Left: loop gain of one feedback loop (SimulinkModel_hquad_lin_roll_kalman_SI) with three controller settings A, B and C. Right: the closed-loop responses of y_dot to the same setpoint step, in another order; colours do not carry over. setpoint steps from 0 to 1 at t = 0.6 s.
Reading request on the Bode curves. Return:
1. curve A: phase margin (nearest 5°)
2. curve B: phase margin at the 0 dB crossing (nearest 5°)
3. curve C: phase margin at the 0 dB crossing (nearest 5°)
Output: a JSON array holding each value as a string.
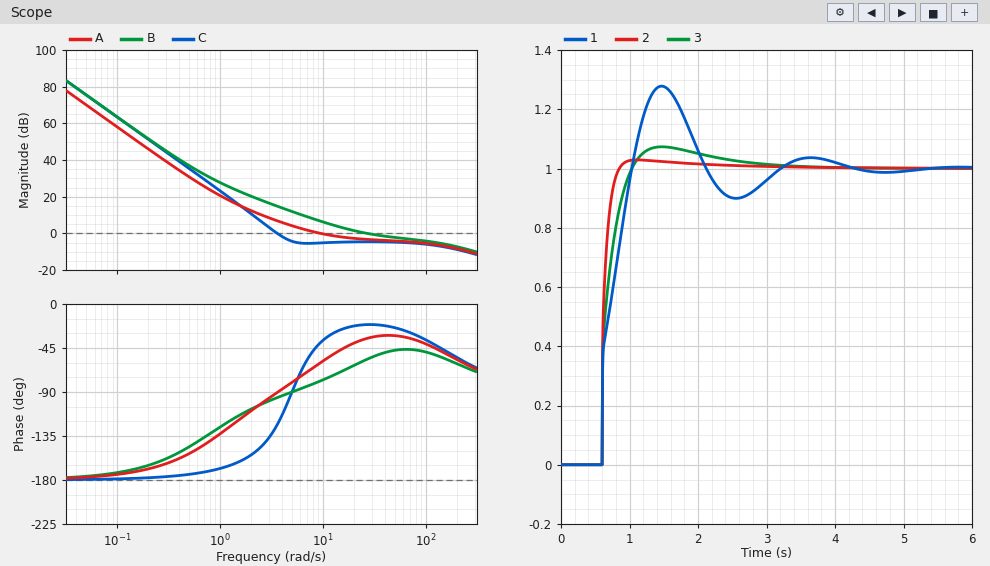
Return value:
["120°", "125°", "55°"]
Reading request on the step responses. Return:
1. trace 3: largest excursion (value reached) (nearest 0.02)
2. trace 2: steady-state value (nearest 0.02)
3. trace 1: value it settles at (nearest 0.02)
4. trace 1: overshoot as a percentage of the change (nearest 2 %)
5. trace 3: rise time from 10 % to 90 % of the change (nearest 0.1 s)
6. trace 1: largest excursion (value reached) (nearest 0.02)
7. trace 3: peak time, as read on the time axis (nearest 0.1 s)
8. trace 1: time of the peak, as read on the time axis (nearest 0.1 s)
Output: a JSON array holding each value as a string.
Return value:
["1.08", "1.00", "1.00", "28 %", "0.3 s", "1.28", "1.5 s", "1.5 s"]
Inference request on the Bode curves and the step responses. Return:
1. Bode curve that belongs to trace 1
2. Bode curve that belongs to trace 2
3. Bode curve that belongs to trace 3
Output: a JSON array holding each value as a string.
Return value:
["C", "B", "A"]
